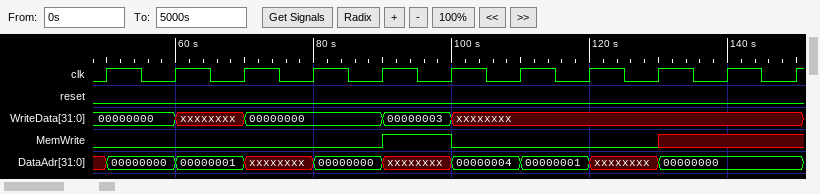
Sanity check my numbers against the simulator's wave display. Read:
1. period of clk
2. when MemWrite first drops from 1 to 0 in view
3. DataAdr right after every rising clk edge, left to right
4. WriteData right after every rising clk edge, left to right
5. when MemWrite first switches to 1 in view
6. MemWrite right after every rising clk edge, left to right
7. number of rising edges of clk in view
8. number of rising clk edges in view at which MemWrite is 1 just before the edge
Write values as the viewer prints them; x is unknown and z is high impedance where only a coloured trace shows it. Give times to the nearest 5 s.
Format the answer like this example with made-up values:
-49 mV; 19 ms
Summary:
10 s; 100 s; 00000000, 00000001, xxxxxxxx, 00000000, xxxxxxxx, 00000004, 00000001, xxxxxxxx, 00000000, 00000000, 00000000; 00000000, xxxxxxxx, 00000000, 00000000, 00000003, xxxxxxxx, xxxxxxxx, xxxxxxxx, xxxxxxxx, xxxxxxxx, xxxxxxxx; 90 s; 0 0 0 0 1 0 0 0 x x x; 11; 1
